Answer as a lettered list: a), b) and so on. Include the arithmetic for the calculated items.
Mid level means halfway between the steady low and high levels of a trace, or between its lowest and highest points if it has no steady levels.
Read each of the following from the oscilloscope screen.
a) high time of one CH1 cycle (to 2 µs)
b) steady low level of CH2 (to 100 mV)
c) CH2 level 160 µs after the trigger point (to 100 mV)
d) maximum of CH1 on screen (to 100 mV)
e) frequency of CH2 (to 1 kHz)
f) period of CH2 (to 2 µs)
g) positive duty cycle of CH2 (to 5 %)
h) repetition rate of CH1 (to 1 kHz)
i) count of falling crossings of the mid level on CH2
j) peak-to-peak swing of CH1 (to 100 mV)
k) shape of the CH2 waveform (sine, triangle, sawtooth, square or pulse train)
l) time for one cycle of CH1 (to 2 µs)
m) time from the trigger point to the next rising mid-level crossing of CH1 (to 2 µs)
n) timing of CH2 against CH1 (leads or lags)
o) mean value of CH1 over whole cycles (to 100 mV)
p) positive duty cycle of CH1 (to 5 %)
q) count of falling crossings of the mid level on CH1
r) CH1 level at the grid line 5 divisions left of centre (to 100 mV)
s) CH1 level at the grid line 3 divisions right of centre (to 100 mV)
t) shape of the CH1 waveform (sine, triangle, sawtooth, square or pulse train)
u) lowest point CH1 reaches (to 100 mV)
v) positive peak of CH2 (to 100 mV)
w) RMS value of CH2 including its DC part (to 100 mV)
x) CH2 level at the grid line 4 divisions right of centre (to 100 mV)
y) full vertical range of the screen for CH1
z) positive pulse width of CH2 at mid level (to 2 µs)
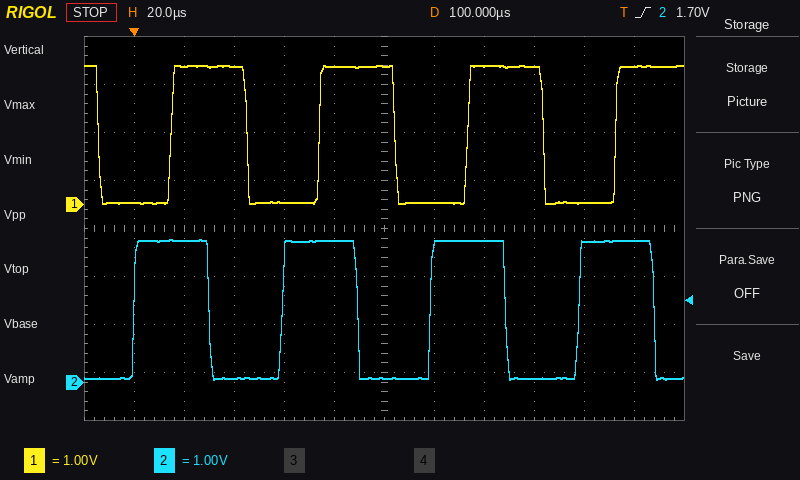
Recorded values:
a) 30 µs
b) 100 mV
c) 100 mV
d) 2.9 V
e) 1 / 60 µs ≈ 17 kHz
f) 60 µs
g) 30 µs / 60 µs ≈ 50 %
h) 1 / 60 µs ≈ 17 kHz
i) 4
j) 2.9 V − (0.0 V) = 2.9 V
k) square
l) 60 µs
m) 14 µs
n) leads
o) 0.0 V + 0.5 × (2.9 V − (0.0 V)) ≈ 1.5 V
p) 30 µs / 60 µs ≈ 50 %
q) 4
r) 0.0 V
s) 2.9 V
t) square
u) 0.0 V
v) 3.0 V
w) √(0.5 × (3.0 V)² + 0.5 × (100 mV)²) ≈ 2.1 V
x) 2.9 V
y) 8 V
z) 30 µs
